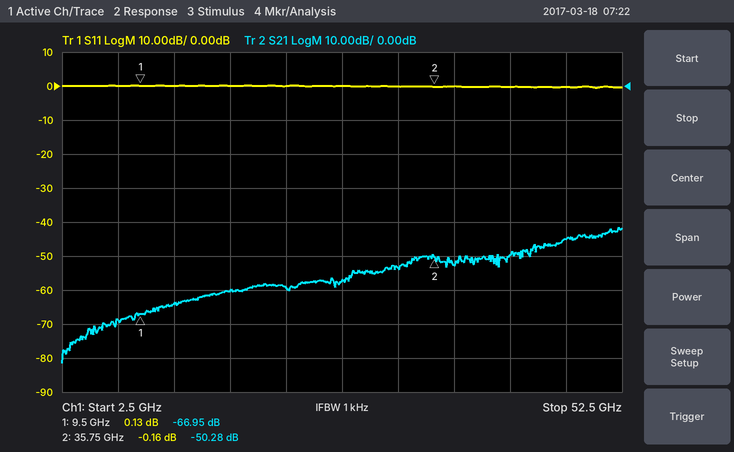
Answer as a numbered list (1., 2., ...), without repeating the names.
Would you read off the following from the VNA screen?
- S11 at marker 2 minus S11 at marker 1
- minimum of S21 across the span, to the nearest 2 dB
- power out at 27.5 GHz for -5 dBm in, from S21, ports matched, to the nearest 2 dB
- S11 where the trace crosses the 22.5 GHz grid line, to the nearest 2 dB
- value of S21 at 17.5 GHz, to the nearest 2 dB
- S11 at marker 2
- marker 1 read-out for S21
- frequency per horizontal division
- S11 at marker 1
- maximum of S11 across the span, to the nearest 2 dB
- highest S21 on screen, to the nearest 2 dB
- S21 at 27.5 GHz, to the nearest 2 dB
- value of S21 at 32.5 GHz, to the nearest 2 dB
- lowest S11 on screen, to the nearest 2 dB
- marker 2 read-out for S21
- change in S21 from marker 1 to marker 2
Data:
1. -0.29 dB
2. -82 dB
3. -62 dBm
4. 0 dB
5. -60 dB
6. -0.16 dB
7. -66.95 dB
8. 5 GHz
9. 0.13 dB
10. 0 dB
11. -42 dB
12. -58 dB
13. -54 dB
14. 0 dB
15. -50.28 dB
16. 16.67 dB
